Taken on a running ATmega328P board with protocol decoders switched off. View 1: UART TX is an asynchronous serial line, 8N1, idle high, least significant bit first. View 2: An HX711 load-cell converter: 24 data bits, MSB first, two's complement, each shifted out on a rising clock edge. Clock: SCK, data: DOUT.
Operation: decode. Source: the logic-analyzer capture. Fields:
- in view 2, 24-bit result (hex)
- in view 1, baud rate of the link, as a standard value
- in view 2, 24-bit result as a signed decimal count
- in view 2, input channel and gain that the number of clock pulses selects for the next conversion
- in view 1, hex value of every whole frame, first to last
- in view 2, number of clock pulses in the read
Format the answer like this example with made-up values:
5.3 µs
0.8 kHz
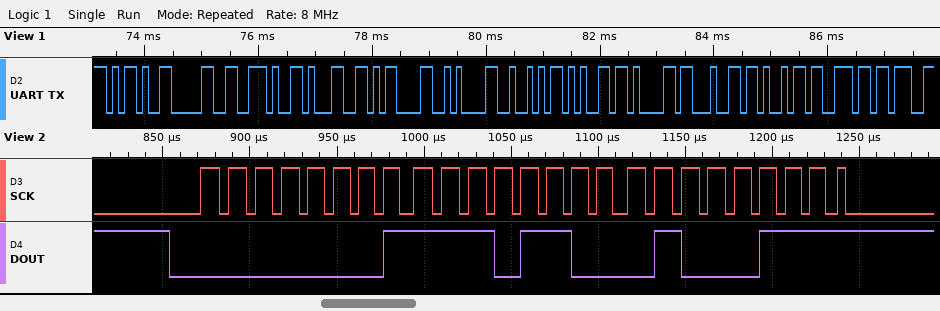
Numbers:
0x01EC47
9600 baud
126023
channel A, gain 128
0x2D 0x30 0x2E 0x31 0x0D 0x0A 0x52 0x65 0x61 0x64 0x69 0x6E
25
